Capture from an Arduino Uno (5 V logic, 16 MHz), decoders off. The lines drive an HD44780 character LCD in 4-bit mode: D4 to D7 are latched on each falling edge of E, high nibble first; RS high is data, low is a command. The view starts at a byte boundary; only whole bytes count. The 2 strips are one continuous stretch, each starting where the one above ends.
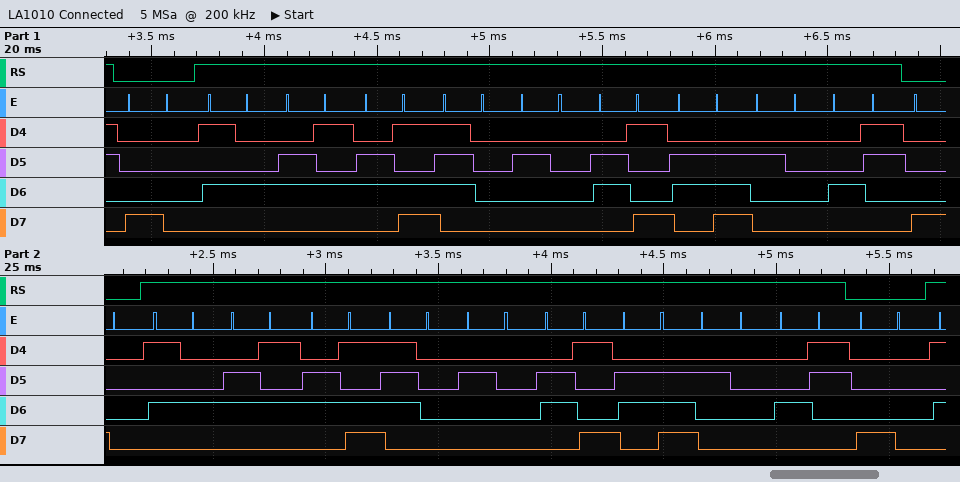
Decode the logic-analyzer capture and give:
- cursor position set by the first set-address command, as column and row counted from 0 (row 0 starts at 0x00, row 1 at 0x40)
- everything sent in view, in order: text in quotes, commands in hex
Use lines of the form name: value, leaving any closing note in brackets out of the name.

cursor position set by the first set-address command, as column and row counted from 0: column 0, row 0
everything sent in view, in order: text in quotes, commands in hex: 0x80 "Temp in C" 0x80 "Temp in C" 0x80
